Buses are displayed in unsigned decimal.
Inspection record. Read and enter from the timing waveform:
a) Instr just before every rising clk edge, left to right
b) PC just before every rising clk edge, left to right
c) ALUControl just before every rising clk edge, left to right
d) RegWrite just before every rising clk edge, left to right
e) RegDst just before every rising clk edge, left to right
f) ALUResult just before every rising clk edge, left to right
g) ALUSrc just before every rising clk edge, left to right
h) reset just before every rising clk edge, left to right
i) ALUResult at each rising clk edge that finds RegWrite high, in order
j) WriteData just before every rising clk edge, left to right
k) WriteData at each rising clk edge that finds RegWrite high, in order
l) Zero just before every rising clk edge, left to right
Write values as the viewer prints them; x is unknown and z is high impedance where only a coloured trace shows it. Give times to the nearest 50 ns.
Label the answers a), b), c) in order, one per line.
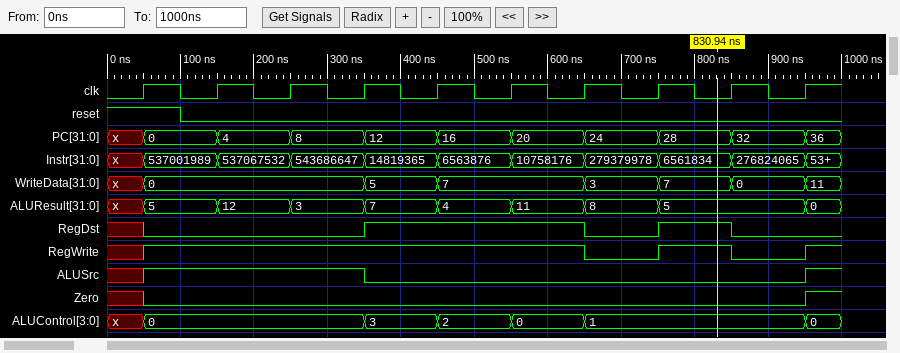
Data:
a) x, 537001989, 537067532, 543686647, 14819365, 6563876, 10758176, 279379978, 6561834, 276824065
b) x, 0, 4, 8, 12, 16, 20, 24, 28, 32
c) x, 0, 0, 0, 3, 2, 0, 1, 1, 1
d) x 1 1 1 1 1 1 0 1 0
e) x 0 0 0 1 1 1 0 1 0
f) x, 5, 12, 3, 7, 4, 11, 8, 5, 5
g) x 1 1 1 0 0 0 0 0 0
h) 1 0 0 0 0 0 0 0 0 0
i) 5, 12, 3, 7, 4, 11, 5
j) x, 0, 0, 0, 5, 7, 7, 3, 7, 0
k) 0, 0, 0, 5, 7, 7, 7
l) x 0 0 0 0 0 0 0 0 0
